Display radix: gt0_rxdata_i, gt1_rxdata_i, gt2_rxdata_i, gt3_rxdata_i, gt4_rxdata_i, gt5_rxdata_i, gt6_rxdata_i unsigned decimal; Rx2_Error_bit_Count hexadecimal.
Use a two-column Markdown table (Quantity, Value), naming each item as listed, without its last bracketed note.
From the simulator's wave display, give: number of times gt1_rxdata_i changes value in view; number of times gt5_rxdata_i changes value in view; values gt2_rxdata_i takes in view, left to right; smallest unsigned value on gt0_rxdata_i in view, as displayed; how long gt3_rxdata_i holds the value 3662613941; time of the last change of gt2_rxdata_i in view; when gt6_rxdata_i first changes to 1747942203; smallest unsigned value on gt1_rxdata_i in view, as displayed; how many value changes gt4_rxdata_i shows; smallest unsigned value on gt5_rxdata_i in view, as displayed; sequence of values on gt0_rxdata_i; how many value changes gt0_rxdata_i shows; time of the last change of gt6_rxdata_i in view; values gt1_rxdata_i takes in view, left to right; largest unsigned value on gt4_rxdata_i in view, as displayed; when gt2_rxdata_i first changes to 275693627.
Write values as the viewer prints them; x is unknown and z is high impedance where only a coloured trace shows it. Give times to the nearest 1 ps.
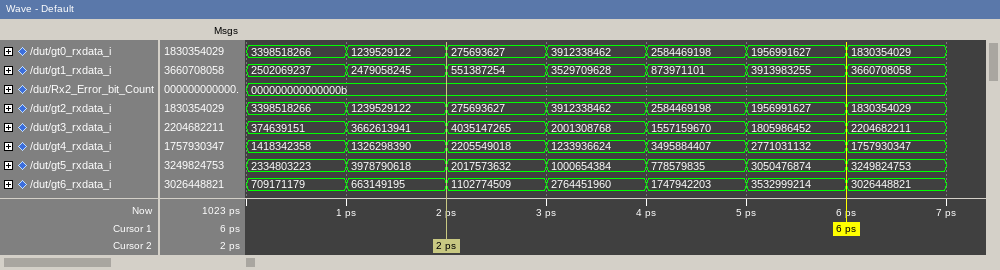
| Quantity | Value |
|---|---|
| number of times gt1_rxdata_i changes value in view | 6 |
| number of times gt5_rxdata_i changes value in view | 6 |
| values gt2_rxdata_i takes in view, left to right | 3398518266, 1239529122, 275693627, 3912338462, 2584469198, 1956991627, 1830354029 |
| smallest unsigned value on gt0_rxdata_i in view, as displayed | 275693627 |
| how long gt3_rxdata_i holds the value 3662613941 | 1 ps |
| time of the last change of gt2_rxdata_i in view | 6 ps |
| when gt6_rxdata_i first changes to 1747942203 | 4 ps |
| smallest unsigned value on gt1_rxdata_i in view, as displayed | 551387254 |
| how many value changes gt4_rxdata_i shows | 6 |
| smallest unsigned value on gt5_rxdata_i in view, as displayed | 778579835 |
| sequence of values on gt0_rxdata_i | 3398518266, 1239529122, 275693627, 3912338462, 2584469198, 1956991627, 1830354029 |
| how many value changes gt0_rxdata_i shows | 6 |
| time of the last change of gt6_rxdata_i in view | 6 ps |
| values gt1_rxdata_i takes in view, left to right | 2502069237, 2479058245, 551387254, 3529709628, 873971101, 3913983255, 3660708058 |
| largest unsigned value on gt4_rxdata_i in view, as displayed | 3495884407 |
| when gt2_rxdata_i first changes to 275693627 | 2 ps |
